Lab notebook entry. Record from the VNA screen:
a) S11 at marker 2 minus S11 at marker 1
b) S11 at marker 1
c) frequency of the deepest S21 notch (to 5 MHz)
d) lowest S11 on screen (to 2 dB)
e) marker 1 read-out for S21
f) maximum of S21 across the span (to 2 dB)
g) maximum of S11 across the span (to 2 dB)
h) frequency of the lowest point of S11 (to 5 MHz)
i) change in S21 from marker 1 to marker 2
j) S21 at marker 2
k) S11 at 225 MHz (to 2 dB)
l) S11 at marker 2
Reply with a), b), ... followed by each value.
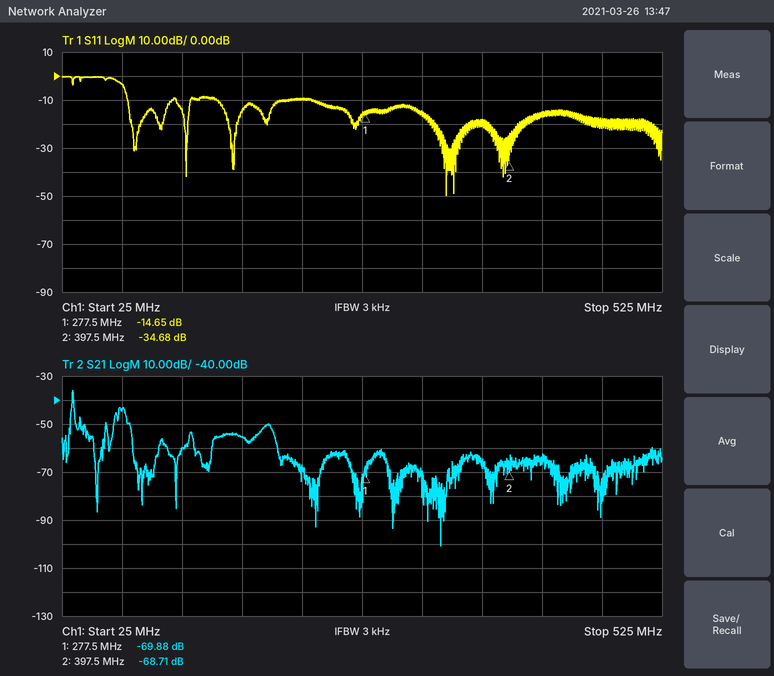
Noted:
a) -20.03 dB
b) -14.65 dB
c) 340 MHz
d) -50 dB
e) -69.88 dB
f) -36 dB
g) 0 dB
h) 345 MHz
i) 1.17 dB
j) -68.71 dB
k) -10 dB
l) -34.68 dB
